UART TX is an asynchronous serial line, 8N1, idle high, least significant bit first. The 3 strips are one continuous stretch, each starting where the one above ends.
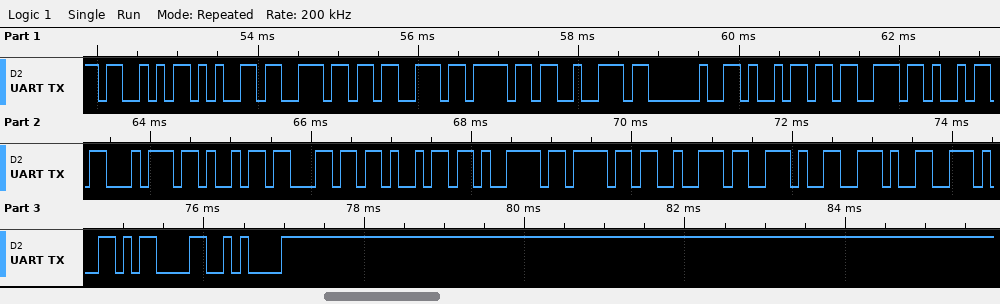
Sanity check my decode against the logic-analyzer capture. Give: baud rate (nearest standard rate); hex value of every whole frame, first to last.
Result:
9600 baud
53 65 6E 73 6F 72 20 69 73 69 74 69 6C 69 79 6F 72 2E 2E 2E 0D 0A
